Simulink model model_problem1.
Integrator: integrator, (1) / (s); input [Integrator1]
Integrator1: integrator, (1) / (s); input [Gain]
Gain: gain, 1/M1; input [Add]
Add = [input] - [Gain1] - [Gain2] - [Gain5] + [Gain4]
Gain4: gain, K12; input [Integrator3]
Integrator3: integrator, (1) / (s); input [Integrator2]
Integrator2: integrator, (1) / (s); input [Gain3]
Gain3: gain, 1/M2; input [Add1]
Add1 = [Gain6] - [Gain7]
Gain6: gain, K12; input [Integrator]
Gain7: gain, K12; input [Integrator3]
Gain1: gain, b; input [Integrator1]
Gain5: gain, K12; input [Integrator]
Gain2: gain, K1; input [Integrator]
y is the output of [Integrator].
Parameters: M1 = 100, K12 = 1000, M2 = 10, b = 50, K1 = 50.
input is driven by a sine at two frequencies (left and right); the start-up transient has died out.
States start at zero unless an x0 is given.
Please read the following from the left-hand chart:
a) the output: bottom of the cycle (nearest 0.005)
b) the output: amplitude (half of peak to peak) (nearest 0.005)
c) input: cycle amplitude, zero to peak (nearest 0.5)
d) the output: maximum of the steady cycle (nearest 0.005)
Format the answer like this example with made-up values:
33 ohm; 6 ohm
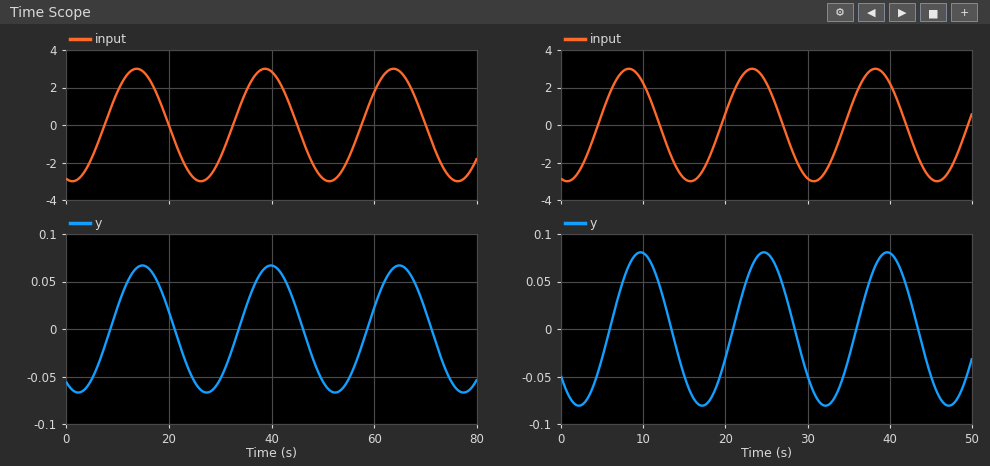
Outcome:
-0.065; 0.065; 3.0; 0.065
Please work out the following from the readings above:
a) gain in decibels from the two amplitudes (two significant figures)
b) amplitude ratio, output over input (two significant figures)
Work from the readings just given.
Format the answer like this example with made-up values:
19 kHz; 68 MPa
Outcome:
-33 dB; 0.022
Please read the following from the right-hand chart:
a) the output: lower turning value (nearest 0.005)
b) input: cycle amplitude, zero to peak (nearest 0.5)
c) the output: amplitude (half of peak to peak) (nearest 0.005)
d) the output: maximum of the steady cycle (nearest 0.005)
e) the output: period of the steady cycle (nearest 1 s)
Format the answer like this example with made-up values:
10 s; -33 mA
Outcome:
-0.080; 3.0; 0.080; 0.080; 15 s
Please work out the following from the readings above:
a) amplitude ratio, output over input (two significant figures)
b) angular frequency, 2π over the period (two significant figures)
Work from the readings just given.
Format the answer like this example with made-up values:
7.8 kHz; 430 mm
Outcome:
0.027; 0.42 rad/s
